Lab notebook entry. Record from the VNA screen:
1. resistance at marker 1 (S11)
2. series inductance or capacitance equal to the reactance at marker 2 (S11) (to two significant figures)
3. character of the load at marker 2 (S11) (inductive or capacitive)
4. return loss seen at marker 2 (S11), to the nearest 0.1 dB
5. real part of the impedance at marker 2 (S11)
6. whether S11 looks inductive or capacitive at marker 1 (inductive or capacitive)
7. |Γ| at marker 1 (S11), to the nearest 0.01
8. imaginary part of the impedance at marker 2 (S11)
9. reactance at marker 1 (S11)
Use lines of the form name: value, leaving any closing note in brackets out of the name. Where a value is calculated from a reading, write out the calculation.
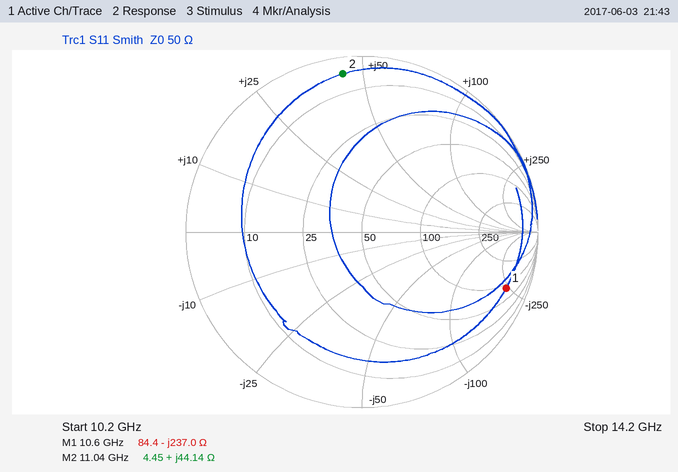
resistance at marker 1: 84.4 Ω
series inductance or capacitance equal to the reactance at marker 2 (S11): L = 44.14 Ω/(2π × 11.04 GHz) ≈ 636 pH, so 640 pH to two significant figures
character of the load at marker 2 (S11): inductive
return loss seen at marker 2 (S11), to the nearest 0.1 dB: 0.9 dB
real part of the impedance at marker 2: 4.45 Ω
whether S11 looks inductive or capacitive at marker 1: capacitive
|Γ| at marker 1 (S11), to the nearest 0.01: 0.88
imaginary part of the impedance at marker 2: +44.14 Ω
reactance at marker 1: -237.0 Ω
